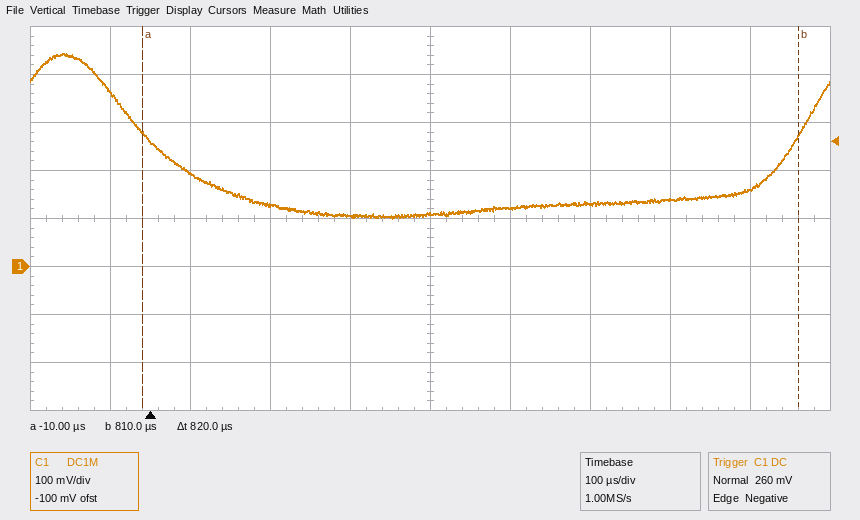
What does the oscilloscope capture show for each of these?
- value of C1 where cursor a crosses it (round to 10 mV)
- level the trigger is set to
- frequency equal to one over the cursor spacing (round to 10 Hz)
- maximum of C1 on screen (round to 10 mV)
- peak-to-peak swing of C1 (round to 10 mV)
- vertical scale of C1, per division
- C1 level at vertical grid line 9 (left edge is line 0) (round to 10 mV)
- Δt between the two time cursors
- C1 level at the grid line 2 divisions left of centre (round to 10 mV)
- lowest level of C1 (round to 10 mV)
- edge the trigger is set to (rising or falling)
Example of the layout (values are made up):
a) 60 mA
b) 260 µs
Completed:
a) 280 mV
b) 260 mV
c) 1.22 kHz
d) 440 mV
e) 340 mV
f) 100 mV
g) 160 mV
h) 820 µs
i) 130 mV
j) 100 mV
k) falling
